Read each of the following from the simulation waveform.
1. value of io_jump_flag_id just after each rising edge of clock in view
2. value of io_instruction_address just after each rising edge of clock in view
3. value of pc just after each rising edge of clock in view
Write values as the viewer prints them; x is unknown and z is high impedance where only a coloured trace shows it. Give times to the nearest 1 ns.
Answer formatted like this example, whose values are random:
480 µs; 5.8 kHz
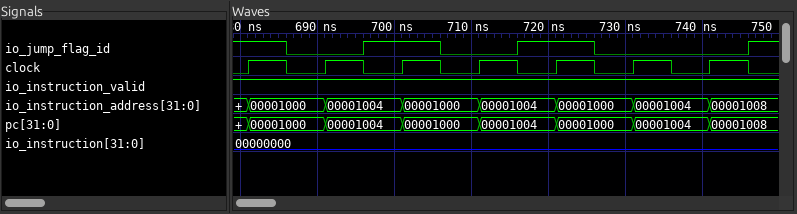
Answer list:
1 0 1 0 1 0 0; 00001000, 00001004, 00001000, 00001004, 00001000, 00001004, 00001008; 00001000, 00001004, 00001000, 00001004, 00001000, 00001004, 00001008
